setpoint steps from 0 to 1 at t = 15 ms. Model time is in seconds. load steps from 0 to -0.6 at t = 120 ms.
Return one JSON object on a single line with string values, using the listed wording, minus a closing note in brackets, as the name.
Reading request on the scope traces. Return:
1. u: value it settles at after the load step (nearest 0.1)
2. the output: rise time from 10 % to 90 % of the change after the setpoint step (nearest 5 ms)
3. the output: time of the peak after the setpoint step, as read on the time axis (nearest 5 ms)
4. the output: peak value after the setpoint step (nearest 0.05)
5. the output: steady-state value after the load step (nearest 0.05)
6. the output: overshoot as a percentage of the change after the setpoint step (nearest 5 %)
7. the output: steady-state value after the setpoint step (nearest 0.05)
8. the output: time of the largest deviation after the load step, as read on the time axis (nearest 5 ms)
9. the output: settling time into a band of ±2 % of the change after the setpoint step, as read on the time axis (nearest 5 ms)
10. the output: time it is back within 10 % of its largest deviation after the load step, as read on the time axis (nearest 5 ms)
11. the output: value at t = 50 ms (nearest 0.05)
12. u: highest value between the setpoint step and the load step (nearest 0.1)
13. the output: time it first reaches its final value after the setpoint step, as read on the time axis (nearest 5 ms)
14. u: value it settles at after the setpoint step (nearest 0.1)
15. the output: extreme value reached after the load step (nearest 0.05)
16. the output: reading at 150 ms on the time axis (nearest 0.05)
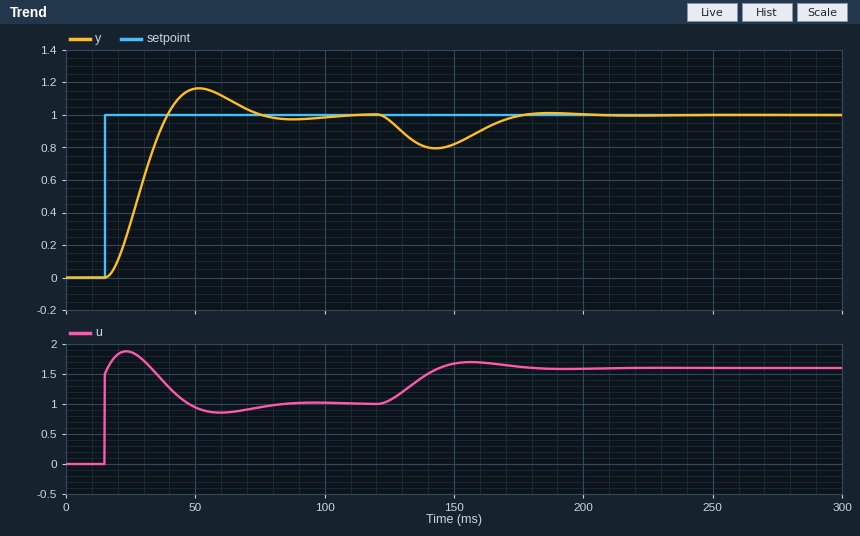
{"u: value it settles at after the load step": "1.6", "the output: rise time from 10 % to 90 % of the change after the setpoint step": "15 ms", "the output: time of the peak after the setpoint step, as read on the time axis": "50 ms", "the output: peak value after the setpoint step": "1.15", "the output: steady-state value after the load step": "1.00", "the output: overshoot as a percentage of the change after the setpoint step": "15 %", "the output: steady-state value after the setpoint step": "1.00", "the output: time of the largest deviation after the load step, as read on the time axis": "145 ms", "the output: settling time into a band of ±2 % of the change after the setpoint step, as read on the time axis": "95 ms", "the output: time it is back within 10 % of its largest deviation after the load step, as read on the time axis": "170 ms", "the output: value at t = 50 ms": "1.15", "u: highest value between the setpoint step and the load step": "1.9", "the output: time it first reaches its final value after the setpoint step, as read on the time axis": "40 ms", "u: value it settles at after the setpoint step": "1.0", "the output: extreme value reached after the load step": "0.80", "the output: reading at 150 ms on the time axis": "0.80"}
